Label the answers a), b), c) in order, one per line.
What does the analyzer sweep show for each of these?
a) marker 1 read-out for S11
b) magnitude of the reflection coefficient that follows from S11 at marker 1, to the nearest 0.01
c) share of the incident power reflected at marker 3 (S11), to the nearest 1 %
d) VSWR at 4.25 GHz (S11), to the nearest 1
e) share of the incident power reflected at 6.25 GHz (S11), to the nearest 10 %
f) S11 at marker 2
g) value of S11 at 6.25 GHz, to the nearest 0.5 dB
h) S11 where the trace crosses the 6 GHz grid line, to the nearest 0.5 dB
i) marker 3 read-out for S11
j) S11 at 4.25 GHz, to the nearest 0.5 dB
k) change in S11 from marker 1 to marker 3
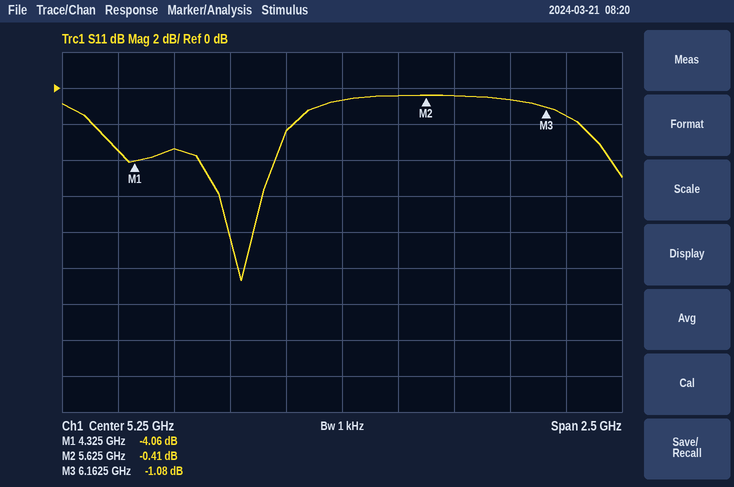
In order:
a) -4.06 dB
b) 0.63
c) 78 %
d) 5
e) 70 %
f) -0.41 dB
g) -1.5 dB
h) -0.5 dB
i) -1.08 dB
j) -3.5 dB
k) 2.98 dB
